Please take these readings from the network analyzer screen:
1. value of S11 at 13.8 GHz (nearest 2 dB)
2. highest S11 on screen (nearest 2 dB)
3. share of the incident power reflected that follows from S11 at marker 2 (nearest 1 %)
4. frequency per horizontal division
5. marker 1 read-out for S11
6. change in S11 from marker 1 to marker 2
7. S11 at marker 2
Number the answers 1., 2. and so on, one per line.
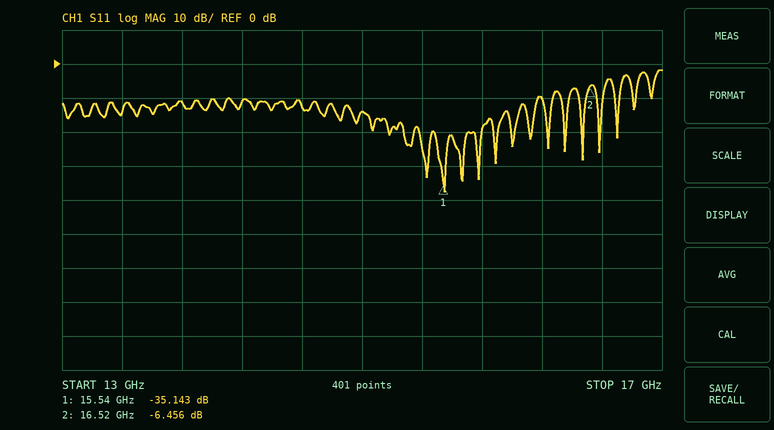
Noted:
1. -12 dB
2. -2 dB
3. 23 %
4. 400 MHz
5. -35.143 dB
6. 28.687 dB
7. -6.456 dB
